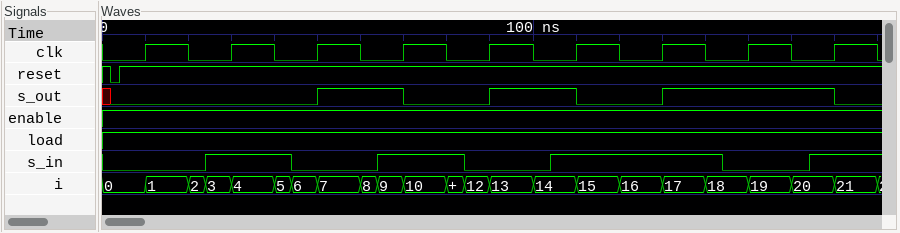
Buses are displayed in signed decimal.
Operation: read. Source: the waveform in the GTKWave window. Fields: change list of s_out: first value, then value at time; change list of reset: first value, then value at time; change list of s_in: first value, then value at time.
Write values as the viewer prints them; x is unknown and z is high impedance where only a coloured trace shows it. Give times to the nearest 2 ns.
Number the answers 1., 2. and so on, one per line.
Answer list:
1. x, 0 at 2 ns, 1 at 50 ns, 0 at 70 ns, 1 at 90 ns, 0 at 110 ns, 1 at 130 ns, 0 at 170 ns
2. 1, 0 at 2 ns, 1 at 4 ns
3. 0, 1 at 24 ns, 0 at 44 ns, 1 at 64 ns, 0 at 84 ns, 1 at 104 ns, 0 at 144 ns, 1 at 164 ns
